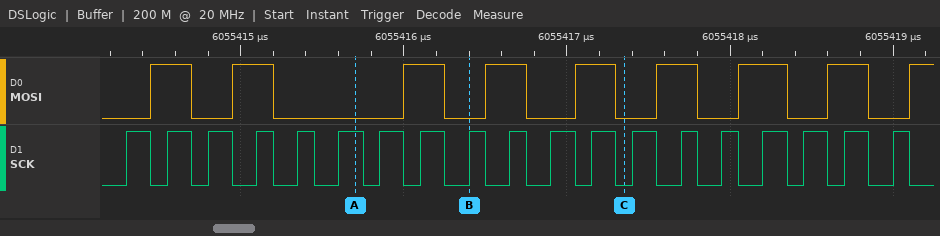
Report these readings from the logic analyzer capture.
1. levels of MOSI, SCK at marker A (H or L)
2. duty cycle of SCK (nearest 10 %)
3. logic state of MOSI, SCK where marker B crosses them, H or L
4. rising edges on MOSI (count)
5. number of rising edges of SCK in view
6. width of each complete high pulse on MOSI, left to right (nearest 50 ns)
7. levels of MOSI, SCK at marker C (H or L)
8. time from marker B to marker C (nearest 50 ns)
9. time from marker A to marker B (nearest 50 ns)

MOSI=L, SCK=H
50 %
MOSI=L, SCK=H
9
19
250 ns, 250 ns, 250 ns, 250 ns, 250 ns, 250 ns, 300 ns, 250 ns
MOSI=L, SCK=L
950 ns
700 ns
